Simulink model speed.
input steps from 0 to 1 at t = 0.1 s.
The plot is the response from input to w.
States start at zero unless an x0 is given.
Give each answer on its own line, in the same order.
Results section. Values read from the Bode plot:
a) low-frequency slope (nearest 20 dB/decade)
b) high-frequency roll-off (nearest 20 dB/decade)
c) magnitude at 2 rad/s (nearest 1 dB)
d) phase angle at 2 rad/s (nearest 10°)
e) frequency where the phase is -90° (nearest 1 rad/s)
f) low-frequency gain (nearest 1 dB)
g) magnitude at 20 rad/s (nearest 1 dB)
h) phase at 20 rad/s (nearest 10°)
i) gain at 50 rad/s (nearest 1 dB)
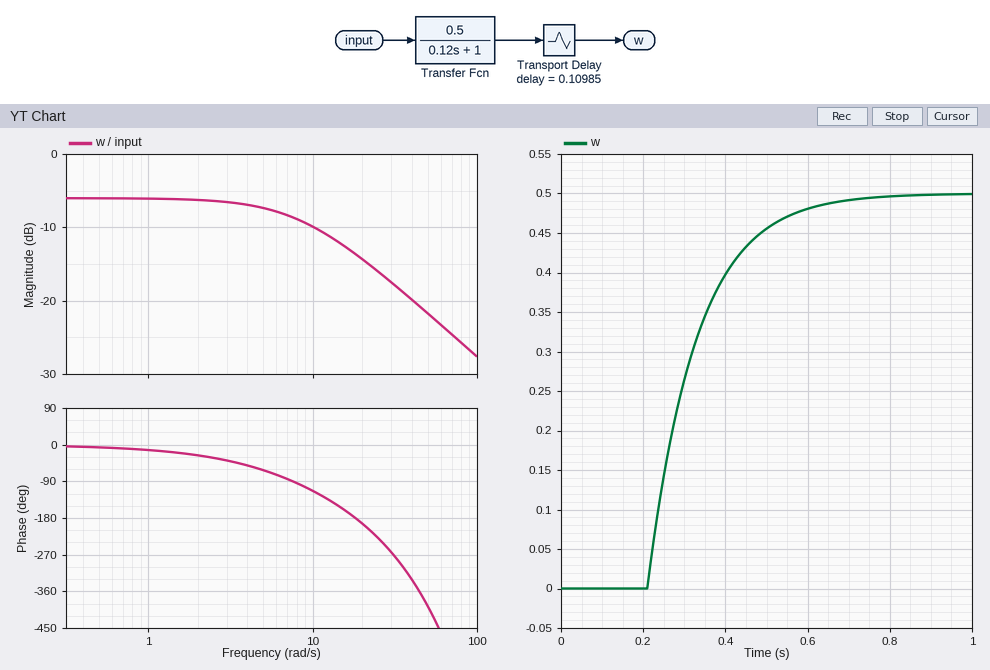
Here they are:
0 dB/decade
-20 dB/decade
-6 dB
-30°
8 rad/s
-6 dB
-14 dB
-190°
-22 dB
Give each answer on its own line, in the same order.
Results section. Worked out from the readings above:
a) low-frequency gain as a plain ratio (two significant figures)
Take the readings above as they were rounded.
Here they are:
0.50
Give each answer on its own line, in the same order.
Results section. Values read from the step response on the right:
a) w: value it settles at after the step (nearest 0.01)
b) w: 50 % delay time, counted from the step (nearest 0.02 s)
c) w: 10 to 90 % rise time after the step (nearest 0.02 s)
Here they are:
0.50
0.20 s
0.26 s
